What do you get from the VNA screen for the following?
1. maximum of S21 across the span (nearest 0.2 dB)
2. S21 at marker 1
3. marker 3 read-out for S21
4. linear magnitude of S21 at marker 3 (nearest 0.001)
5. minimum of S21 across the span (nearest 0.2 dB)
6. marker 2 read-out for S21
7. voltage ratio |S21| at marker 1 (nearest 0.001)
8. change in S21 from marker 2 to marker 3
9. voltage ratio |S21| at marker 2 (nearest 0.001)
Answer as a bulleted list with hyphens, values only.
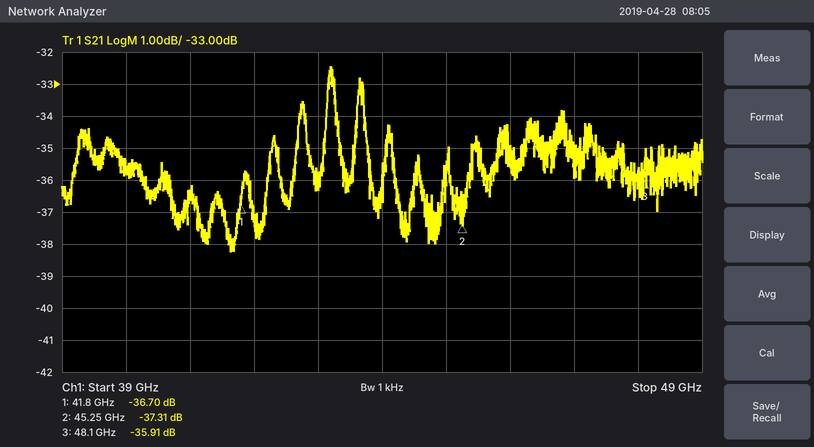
- -32.4 dB
- -36.70 dB
- -35.91 dB
- 0.016
- -38.2 dB
- -37.31 dB
- 0.015
- 1.40 dB
- 0.014
